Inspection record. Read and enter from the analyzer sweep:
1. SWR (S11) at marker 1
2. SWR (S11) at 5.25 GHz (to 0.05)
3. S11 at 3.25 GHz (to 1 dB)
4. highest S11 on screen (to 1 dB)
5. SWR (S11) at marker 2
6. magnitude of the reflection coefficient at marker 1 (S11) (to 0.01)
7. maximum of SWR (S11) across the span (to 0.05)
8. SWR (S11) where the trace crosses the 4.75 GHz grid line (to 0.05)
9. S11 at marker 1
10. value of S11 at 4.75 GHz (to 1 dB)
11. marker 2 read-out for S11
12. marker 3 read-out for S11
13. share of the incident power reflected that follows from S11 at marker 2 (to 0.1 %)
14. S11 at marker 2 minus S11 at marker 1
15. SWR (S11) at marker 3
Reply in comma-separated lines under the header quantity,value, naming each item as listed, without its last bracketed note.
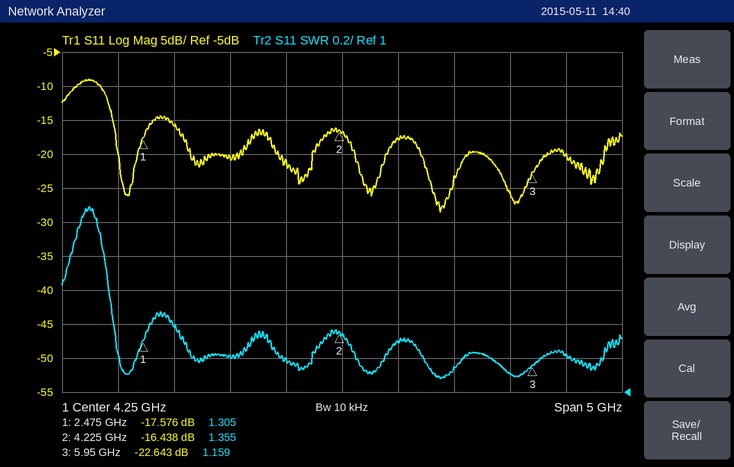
quantity,value
SWR (S11) at marker 1,1.305
SWR (S11) at 5.25 GHz,1.15
S11 at 3.25 GHz,-20 dB
highest S11 on screen,-9 dB
SWR (S11) at marker 2,1.355
magnitude of the reflection coefficient at marker 1 (S11),0.13
maximum of SWR (S11) across the span,2.10
SWR (S11) where the trace crosses the 4.75 GHz grid line,1.30
S11 at marker 1,-17.576 dB
value of S11 at 4.75 GHz,-18 dB
marker 2 read-out for S11,-16.438 dB
marker 3 read-out for S11,-22.643 dB
share of the incident power reflected that follows from S11 at marker 2,2.3 %
S11 at marker 2 minus S11 at marker 1,1.138 dB
SWR (S11) at marker 3,1.159
